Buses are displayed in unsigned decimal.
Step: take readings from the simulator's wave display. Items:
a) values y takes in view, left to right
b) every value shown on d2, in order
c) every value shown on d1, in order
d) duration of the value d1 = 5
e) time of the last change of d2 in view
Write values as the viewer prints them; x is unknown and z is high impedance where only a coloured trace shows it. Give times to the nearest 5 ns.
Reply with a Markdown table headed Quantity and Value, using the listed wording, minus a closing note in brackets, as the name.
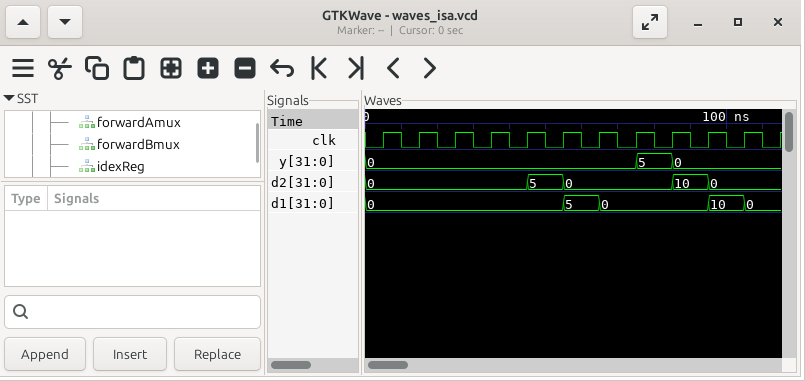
| Quantity | Value |
|---|---|
| values y takes in view, left to right | 0, 5, 0 |
| every value shown on d2, in order | 0, 5, 0, 10, 0 |
| every value shown on d1, in order | 0, 5, 0, 10, 0 |
| duration of the value d1 = 5 | 10 ns |
| time of the last change of d2 in view | 95 ns |
